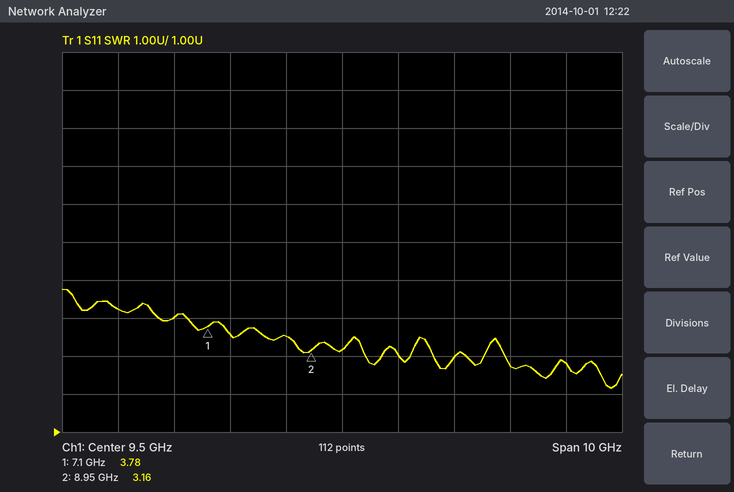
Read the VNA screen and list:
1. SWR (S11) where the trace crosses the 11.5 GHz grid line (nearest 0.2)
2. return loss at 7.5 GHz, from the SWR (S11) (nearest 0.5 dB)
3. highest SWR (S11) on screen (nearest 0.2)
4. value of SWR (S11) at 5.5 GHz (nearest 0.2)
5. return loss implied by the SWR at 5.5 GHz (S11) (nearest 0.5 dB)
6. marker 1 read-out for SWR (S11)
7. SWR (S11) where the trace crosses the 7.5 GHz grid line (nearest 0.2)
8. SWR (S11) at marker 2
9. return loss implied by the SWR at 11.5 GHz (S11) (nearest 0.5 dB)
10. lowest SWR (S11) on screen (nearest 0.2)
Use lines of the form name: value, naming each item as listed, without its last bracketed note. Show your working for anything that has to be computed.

SWR (S11) where the trace crosses the 11.5 GHz grid line: 3.0
return loss at 7.5 GHz, from the SWR (S11): −20 log10((3.6 − 1)/(3.6 + 1)) ≈ 5.0 dB
highest SWR (S11) on screen: 4.8
value of SWR (S11) at 5.5 GHz: 4.2
return loss implied by the SWR at 5.5 GHz (S11): −20 log10((4.2 − 1)/(4.2 + 1)) ≈ 4.22 dB, so 4.0 dB to the nearest 0.5 dB
marker 1 read-out for SWR: 3.78
SWR (S11) where the trace crosses the 7.5 GHz grid line: 3.6
SWR (S11) at marker 2: 3.16
return loss implied by the SWR at 11.5 GHz (S11): −20 log10((3 − 1)/(3 + 1)) ≈ 6.0 dB
lowest SWR (S11) on screen: 2.2
